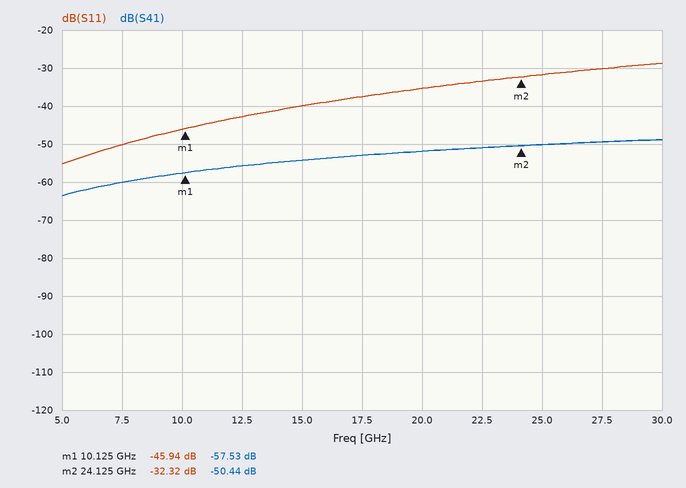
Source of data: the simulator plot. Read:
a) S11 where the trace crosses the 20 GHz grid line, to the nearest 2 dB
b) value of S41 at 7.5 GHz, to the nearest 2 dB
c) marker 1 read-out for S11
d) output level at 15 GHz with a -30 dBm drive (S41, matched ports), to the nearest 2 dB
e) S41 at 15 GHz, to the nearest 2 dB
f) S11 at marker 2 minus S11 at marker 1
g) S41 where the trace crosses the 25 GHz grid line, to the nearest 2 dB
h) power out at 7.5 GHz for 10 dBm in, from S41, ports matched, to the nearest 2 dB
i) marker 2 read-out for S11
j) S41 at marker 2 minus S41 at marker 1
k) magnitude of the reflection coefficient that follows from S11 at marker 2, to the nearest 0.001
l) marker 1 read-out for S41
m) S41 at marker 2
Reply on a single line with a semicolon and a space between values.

-36 dB; -60 dB; -45.94 dB; -84 dBm; -54 dB; 13.62 dB; -50 dB; -50 dBm; -32.32 dB; 7.09 dB; 0.024; -57.53 dB; -50.44 dB
